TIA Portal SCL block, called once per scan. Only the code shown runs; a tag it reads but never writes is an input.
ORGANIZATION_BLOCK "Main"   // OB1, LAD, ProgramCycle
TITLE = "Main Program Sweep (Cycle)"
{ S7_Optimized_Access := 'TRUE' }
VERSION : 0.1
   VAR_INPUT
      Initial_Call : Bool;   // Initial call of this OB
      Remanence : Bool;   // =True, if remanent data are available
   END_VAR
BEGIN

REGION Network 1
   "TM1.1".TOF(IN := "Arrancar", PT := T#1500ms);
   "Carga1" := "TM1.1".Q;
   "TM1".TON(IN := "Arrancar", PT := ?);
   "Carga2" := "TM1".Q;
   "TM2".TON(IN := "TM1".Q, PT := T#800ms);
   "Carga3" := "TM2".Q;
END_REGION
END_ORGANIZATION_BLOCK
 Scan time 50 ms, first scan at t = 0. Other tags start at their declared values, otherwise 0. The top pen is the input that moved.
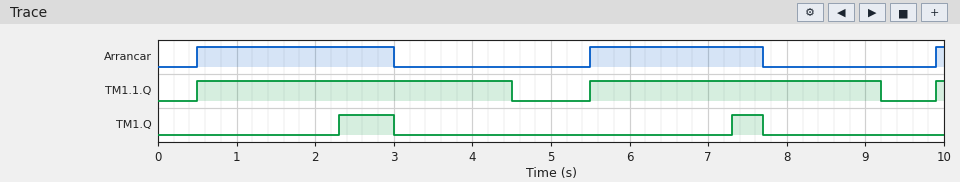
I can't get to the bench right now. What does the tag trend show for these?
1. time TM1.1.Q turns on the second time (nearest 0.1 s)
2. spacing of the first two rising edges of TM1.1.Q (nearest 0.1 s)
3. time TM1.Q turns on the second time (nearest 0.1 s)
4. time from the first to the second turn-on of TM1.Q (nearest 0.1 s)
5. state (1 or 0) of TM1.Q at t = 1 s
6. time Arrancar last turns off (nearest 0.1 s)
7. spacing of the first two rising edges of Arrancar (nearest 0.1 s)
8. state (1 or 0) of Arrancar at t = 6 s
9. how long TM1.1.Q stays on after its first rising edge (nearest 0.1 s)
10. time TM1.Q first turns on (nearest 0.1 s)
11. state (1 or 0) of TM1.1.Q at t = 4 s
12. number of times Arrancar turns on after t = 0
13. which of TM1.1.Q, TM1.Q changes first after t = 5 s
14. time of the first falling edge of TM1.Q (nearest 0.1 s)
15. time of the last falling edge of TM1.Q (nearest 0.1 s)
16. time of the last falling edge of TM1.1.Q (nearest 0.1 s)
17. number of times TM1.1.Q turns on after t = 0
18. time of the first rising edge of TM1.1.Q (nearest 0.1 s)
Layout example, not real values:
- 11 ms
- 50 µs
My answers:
- 5.5 s
- 5.0 s
- 7.3 s
- 5.0 s
- 0
- 7.7 s
- 5.0 s
- 1
- 4.0 s
- 2.3 s
- 1
- 3
- TM1.1.Q
- 3.0 s
- 7.7 s
- 9.2 s
- 3
- 0.5 s
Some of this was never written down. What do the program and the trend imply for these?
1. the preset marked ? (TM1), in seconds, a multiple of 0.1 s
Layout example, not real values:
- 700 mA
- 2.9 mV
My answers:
- 1.8 s
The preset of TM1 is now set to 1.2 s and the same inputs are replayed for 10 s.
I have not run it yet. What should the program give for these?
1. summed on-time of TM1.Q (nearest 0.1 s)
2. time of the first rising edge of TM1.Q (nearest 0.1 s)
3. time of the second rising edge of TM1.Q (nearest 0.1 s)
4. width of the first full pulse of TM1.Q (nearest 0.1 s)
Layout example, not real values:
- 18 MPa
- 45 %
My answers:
- 2.3 s
- 1.7 s
- 6.7 s
- 1.3 s
